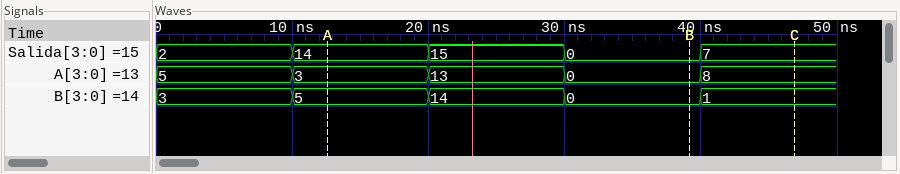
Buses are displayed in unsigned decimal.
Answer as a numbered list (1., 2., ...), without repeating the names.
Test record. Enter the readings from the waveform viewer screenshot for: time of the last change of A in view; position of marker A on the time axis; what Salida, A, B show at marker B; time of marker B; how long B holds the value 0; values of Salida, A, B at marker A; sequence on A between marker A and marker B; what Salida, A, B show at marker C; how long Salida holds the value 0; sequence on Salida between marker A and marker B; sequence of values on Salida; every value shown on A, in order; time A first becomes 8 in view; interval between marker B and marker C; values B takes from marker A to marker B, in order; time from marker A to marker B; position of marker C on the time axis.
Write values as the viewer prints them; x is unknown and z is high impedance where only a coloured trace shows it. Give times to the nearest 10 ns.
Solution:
1. 40 ns
2. 10 ns
3. Salida=0, A=0, B=0
4. 40 ns
5. 10 ns
6. Salida=14, A=3, B=5
7. 3, 13, 0
8. Salida=7, A=8, B=1
9. 10 ns
10. 14, 15, 0
11. 2, 14, 15, 0, 7
12. 5, 3, 13, 0, 8
13. 40 ns
14. 10 ns
15. 5, 14, 0
16. 30 ns
17. 50 ns
